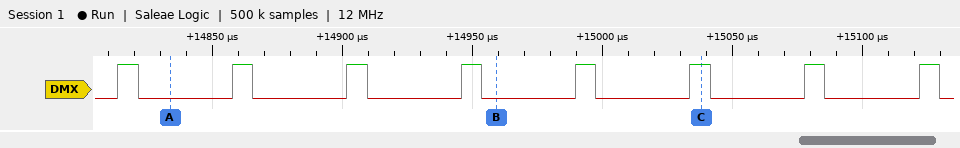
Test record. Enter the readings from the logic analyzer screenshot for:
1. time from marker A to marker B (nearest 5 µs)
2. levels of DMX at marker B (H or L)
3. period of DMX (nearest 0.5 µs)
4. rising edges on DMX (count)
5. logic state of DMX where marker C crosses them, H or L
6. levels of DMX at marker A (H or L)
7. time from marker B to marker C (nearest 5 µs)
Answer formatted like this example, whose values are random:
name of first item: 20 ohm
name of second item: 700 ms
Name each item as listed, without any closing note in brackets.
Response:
time from marker A to marker B: 125 µs
levels of DMX at marker B: DMX=L
period of DMX: 44 µs
rising edges on DMX: 8
logic state of DMX where marker C crosses them, H or L: DMX=H
levels of DMX at marker A: DMX=L
time from marker B to marker C: 80 µs
